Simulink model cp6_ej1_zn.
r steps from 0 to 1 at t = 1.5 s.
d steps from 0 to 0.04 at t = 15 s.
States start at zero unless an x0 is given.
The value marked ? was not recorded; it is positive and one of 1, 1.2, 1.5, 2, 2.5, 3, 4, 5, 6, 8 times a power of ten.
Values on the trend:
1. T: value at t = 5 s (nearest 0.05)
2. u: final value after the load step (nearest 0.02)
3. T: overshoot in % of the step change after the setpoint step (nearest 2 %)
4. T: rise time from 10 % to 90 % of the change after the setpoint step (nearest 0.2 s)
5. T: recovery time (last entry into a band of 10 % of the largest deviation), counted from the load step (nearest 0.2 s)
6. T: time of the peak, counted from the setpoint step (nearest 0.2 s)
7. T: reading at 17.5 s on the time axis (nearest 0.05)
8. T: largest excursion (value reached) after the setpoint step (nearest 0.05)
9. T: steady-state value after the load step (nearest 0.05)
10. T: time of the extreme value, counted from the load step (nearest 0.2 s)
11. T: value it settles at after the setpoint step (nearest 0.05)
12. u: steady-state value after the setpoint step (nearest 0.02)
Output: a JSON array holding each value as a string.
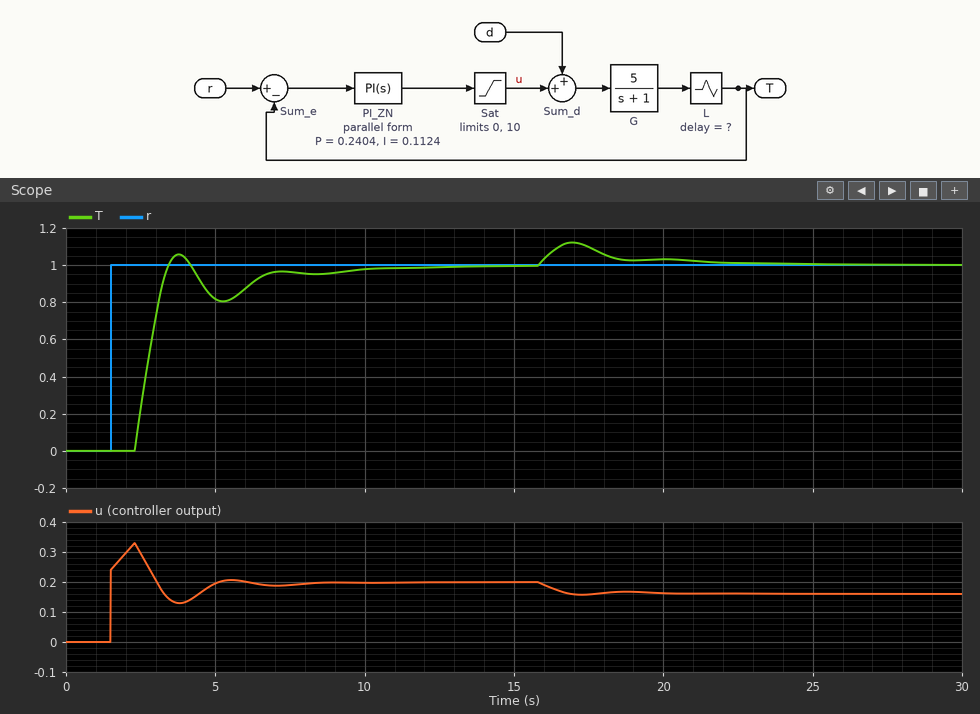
["0.80", "0.16", "6 %", "0.8 s", "7.0 s", "2.2 s", "1.10", "1.05", "1.00", "2.0 s", "1.00", "0.20"]
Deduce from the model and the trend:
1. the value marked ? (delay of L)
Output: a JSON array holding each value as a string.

["0.8"]
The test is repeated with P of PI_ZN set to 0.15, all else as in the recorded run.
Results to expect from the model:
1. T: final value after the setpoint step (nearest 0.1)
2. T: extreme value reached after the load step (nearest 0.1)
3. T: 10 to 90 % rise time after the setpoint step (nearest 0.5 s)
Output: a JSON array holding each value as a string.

["1.0", "1.1", "1.5 s"]
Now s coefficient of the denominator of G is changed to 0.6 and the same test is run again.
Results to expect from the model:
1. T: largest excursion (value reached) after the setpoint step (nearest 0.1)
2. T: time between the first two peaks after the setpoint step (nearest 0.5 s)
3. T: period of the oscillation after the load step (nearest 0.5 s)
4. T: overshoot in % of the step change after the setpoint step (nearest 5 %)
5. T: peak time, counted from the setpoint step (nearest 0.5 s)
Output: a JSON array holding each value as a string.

["1.2", "2.5 s", "2.5 s", "20 %", "2.0 s"]
